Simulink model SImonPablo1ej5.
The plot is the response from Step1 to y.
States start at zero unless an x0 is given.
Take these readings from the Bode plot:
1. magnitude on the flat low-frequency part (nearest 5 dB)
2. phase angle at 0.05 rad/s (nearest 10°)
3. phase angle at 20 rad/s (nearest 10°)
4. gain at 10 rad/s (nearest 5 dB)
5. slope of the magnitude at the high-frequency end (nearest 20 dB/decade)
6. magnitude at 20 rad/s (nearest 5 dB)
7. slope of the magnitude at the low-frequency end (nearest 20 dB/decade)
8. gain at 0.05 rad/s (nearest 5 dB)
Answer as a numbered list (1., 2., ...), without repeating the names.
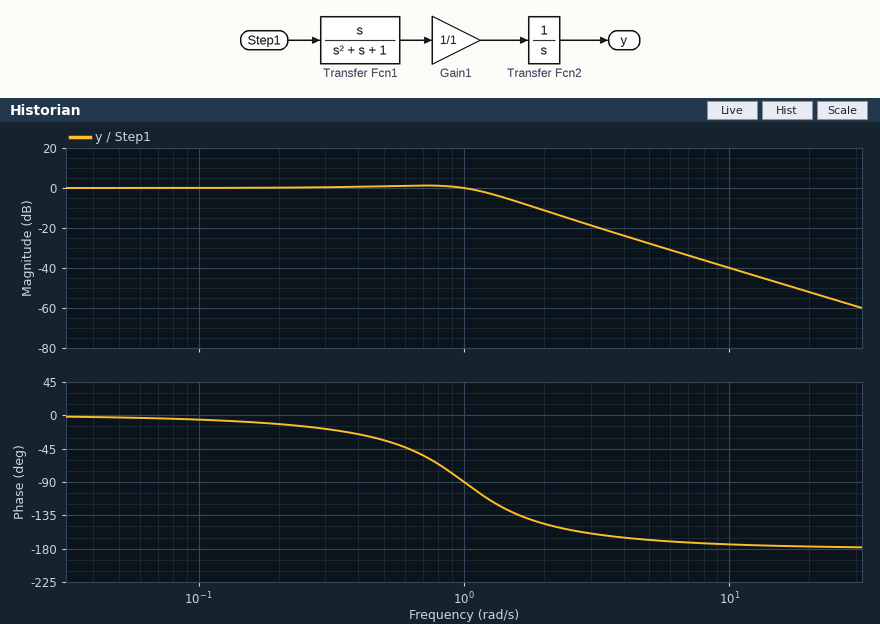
1. 0 dB
2. 0°
3. -180°
4. -40 dB
5. -40 dB/decade
6. -50 dB
7. 0 dB/decade
8. 0 dB
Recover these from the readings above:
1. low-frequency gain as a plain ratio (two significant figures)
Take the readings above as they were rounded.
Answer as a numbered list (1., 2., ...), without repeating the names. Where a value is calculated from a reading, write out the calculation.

1. 10^(0 / 20) = 1.0
